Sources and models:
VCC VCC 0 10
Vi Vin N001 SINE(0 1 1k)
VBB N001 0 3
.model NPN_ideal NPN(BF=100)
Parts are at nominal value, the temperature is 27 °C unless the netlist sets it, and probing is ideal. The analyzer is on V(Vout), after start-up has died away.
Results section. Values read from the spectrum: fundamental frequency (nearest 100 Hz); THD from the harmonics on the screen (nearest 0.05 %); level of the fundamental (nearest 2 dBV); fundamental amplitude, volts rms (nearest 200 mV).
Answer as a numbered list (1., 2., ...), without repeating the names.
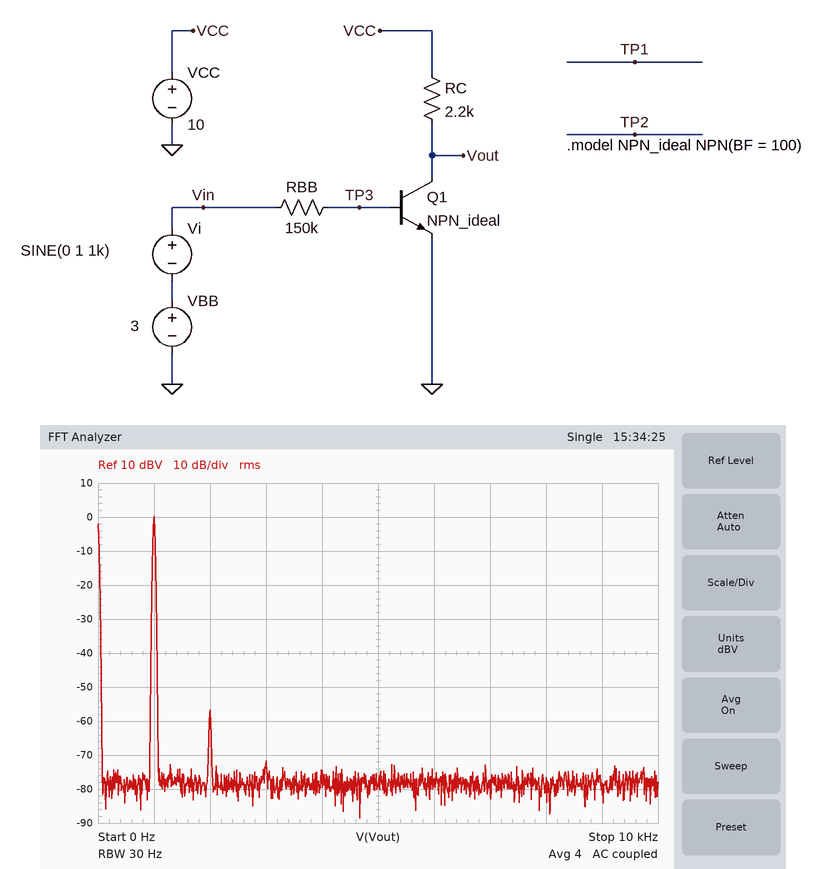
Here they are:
1. 1.0 kHz
2. 0.15 %
3. 0 dBV
4. 1.0 V
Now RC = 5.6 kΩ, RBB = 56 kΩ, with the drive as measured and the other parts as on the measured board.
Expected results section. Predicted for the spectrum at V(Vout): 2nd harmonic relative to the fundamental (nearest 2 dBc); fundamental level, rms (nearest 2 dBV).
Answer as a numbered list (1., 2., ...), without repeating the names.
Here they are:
1. -12 dBc
2. -34 dBV
